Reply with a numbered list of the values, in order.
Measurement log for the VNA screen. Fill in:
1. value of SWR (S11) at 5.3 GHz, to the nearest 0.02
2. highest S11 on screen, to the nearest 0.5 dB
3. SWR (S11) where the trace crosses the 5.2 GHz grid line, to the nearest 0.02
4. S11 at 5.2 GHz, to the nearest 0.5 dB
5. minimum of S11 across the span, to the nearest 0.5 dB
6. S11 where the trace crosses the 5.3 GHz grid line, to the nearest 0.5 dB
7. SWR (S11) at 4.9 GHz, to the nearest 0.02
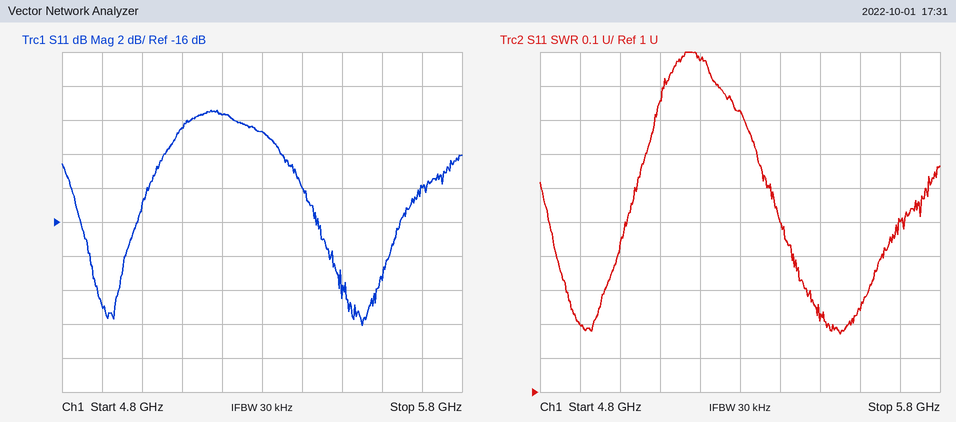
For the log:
1. 1.82
2. -9.5 dB
3. 1.98
4. -9.5 dB
5. -22.0 dB
6. -10.5 dB
7. 1.20
